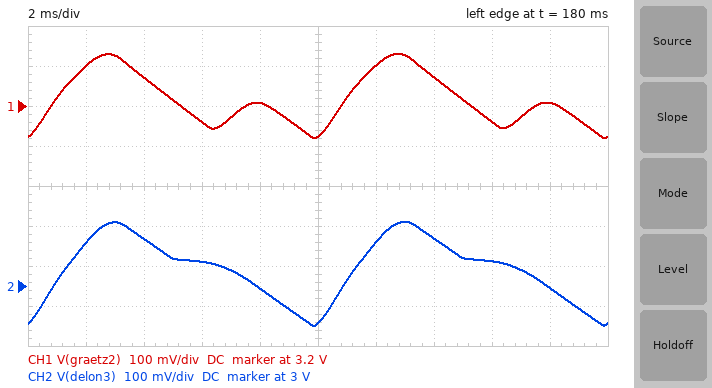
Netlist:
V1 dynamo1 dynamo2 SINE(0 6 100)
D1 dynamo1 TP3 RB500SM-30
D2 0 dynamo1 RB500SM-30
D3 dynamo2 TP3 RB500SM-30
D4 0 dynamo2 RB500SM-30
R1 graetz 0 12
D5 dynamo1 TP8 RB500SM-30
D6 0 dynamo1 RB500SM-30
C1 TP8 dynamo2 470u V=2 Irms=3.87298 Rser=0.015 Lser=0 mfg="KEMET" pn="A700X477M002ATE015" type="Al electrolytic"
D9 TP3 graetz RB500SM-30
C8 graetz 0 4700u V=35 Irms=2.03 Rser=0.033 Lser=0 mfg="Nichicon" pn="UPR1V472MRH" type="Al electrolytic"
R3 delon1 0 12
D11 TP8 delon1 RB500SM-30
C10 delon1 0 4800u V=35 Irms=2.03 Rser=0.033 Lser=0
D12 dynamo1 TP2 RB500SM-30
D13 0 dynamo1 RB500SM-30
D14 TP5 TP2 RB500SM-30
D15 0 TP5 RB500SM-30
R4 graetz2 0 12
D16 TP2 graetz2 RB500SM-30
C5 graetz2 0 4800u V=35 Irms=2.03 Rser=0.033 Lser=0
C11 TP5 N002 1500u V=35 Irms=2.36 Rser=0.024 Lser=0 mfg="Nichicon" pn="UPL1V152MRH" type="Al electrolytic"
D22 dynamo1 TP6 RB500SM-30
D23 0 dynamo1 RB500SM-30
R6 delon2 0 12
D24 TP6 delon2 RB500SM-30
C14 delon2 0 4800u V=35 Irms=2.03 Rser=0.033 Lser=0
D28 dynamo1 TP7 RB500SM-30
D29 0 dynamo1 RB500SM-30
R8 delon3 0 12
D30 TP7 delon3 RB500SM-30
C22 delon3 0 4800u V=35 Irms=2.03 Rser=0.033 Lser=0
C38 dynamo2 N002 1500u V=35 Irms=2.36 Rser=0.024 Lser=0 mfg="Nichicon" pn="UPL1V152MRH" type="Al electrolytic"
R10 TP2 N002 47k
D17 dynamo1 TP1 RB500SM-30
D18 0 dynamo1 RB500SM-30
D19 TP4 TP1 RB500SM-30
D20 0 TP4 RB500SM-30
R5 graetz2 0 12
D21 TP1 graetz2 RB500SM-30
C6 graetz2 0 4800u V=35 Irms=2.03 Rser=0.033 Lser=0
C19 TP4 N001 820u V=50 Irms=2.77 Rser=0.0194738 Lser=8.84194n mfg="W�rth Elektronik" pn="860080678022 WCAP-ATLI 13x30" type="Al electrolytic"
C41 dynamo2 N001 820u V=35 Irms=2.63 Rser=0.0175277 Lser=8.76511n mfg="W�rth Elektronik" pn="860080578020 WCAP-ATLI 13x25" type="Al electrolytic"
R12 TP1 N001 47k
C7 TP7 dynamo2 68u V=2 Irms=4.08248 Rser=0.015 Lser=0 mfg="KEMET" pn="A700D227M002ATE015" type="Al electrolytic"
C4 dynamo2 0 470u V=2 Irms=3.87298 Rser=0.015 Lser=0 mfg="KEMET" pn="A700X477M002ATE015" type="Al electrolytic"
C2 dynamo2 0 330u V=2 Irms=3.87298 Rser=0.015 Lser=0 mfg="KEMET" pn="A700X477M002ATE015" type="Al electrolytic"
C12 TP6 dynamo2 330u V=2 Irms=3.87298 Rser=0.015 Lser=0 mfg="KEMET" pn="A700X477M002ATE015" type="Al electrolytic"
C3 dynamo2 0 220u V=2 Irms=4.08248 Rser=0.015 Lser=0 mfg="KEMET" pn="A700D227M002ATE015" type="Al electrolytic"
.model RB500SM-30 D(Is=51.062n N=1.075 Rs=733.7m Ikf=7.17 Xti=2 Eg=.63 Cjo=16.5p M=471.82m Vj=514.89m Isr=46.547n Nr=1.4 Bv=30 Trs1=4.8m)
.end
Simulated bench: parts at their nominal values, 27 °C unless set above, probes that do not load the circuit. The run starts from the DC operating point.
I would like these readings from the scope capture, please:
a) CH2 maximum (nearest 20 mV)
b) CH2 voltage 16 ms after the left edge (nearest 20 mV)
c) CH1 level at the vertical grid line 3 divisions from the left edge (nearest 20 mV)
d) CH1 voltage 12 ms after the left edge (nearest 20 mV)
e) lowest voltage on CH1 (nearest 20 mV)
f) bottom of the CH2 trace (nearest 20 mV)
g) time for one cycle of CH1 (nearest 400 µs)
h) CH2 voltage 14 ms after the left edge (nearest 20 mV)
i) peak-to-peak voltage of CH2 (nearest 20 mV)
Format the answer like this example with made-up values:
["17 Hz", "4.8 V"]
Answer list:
["3.16 V", "3.06 V", "3.16 V", "3.30 V", "3.12 V", "2.90 V", "10.0 ms", "3.12 V", "260 mV"]
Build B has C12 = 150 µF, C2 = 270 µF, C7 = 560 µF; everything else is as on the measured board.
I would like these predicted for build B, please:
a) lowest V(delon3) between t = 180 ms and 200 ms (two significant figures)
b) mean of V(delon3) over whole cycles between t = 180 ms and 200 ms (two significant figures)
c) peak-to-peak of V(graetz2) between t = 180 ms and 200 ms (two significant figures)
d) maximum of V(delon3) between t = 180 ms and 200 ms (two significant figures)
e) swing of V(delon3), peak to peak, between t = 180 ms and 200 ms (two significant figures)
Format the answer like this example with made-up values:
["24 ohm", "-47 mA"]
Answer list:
["3.7 V", "3.9 V", "230 mV", "4.1 V", "420 mV"]
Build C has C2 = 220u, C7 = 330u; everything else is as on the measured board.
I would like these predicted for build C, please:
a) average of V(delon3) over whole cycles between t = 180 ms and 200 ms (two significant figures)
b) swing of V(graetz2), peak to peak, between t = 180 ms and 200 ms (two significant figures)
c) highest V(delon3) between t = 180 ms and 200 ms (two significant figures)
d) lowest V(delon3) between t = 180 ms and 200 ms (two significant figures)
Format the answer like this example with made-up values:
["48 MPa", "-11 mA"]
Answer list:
["3.4 V", "230 mV", "3.6 V", "3.3 V"]
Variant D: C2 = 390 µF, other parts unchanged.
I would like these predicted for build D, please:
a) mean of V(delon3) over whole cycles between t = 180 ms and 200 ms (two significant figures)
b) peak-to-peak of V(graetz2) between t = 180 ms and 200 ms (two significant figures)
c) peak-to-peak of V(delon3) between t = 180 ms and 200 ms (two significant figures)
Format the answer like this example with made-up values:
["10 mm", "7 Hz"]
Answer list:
["3.1 V", "220 mV", "270 mV"]
